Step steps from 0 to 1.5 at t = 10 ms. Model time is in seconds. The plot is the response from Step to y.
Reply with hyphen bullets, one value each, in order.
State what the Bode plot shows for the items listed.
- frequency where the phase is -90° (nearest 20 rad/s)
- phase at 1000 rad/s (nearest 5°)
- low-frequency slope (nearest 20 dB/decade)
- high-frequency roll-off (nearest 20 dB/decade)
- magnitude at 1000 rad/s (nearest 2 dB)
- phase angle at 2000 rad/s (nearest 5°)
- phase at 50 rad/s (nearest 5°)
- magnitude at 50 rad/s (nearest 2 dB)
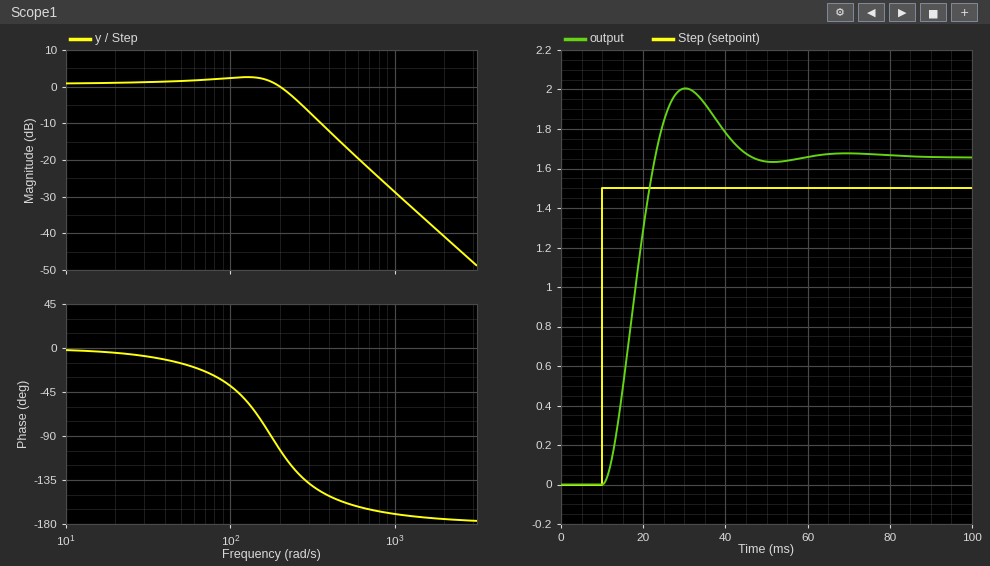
- 180 rad/s
- -170°
- 0 dB/decade
- -40 dB/decade
- -28 dB
- -175°
- -15°
- 2 dB
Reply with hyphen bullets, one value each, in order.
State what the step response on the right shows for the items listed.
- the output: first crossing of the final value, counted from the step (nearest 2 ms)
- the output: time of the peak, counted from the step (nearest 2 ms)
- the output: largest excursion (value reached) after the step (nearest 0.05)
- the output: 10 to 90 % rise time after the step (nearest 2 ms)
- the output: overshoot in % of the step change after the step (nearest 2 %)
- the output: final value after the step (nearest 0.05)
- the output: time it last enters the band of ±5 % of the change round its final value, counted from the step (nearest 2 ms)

- 12 ms
- 20 ms
- 2.00
- 8 ms
- 22 %
- 1.65
- 32 ms
